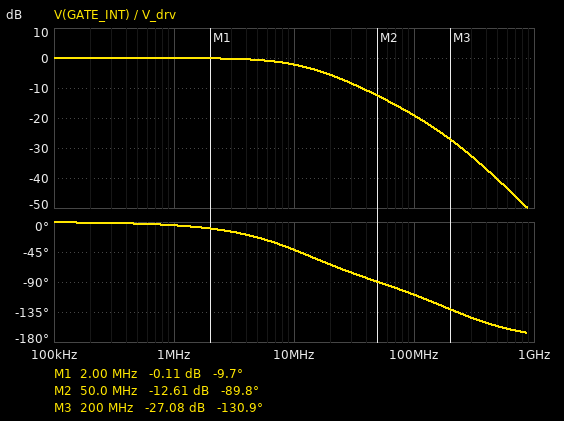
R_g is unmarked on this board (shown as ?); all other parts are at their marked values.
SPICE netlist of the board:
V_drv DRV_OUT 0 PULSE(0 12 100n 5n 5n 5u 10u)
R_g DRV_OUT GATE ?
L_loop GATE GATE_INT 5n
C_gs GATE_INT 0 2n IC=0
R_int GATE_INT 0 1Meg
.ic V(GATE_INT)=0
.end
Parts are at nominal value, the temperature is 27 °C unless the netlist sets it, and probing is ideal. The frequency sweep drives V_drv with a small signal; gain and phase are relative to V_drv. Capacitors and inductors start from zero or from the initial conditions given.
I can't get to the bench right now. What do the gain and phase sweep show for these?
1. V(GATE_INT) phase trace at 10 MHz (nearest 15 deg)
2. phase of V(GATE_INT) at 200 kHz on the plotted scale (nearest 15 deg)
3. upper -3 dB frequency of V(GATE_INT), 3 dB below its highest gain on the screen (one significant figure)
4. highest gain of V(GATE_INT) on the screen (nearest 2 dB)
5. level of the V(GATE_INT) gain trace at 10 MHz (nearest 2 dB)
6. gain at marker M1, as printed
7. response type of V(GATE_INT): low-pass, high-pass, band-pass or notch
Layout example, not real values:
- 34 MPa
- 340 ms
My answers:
- -45 deg
- 0 deg
- 10 MHz
- 0 dB
- -2 dB
- -0.11 dB
- low-pass
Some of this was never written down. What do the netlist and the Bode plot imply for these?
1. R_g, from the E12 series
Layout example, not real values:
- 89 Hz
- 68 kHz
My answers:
- 6.8 Ω
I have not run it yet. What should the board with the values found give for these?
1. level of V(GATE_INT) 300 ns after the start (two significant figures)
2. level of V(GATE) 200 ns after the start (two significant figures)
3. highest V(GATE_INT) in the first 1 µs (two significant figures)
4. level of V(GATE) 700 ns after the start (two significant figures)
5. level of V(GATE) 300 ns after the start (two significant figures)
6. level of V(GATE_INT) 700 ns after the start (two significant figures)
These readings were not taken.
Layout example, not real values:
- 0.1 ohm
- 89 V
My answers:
- 12 V
- 12 V
- 12 V
- 12 V
- 12 V
- 12 V
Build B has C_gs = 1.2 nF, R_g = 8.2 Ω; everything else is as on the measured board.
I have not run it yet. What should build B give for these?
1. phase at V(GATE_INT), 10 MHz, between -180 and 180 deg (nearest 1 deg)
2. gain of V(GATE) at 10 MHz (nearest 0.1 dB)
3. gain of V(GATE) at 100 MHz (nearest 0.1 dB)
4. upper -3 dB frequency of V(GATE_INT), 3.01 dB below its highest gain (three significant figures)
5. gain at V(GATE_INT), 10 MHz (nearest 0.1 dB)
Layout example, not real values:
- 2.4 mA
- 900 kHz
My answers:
- -32 deg
- -1.5 dB
- -13.3 dB
- 17.2 MHz
- -1.3 dB
